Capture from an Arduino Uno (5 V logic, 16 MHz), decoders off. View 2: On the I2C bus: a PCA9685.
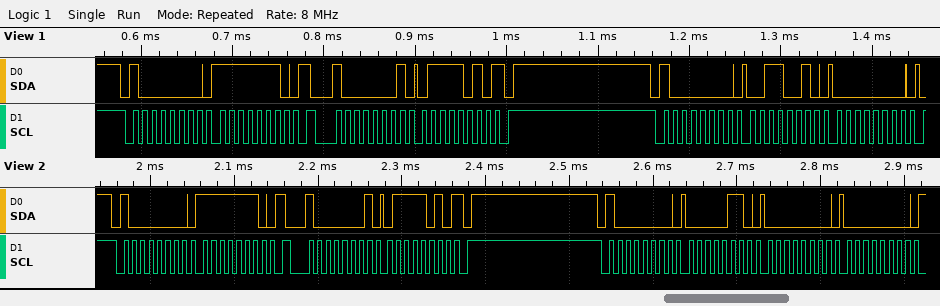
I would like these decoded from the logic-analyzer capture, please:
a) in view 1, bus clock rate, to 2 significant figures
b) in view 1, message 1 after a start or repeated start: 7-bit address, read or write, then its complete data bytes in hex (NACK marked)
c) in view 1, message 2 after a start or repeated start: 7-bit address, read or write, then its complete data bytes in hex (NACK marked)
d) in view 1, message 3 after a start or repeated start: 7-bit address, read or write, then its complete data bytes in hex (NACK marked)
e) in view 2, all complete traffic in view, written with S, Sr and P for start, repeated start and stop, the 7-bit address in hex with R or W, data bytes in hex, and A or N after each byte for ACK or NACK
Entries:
100 kHz
0x40 write: FE
0x40 read: 7A NACK
0x40 write: 32 00
S 40W A FE A Sr 40R A 7A N P S 40W A 06 A 00 A 00 A
